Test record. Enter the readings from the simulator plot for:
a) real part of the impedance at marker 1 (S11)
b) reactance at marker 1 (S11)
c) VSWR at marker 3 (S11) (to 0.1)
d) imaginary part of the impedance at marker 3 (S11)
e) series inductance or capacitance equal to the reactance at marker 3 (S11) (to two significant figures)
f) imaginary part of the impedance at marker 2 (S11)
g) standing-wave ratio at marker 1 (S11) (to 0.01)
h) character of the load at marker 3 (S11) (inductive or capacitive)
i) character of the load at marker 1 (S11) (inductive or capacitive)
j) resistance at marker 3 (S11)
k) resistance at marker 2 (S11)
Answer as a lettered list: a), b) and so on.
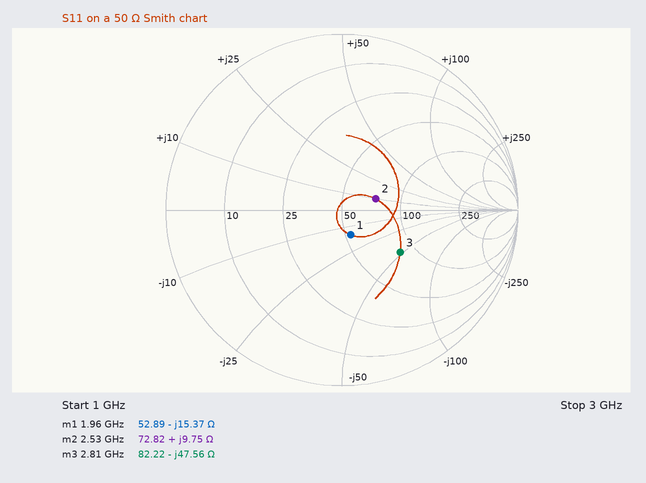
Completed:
a) 52.89 Ω
b) -15.37 Ω
c) 2.4
d) -47.56 Ω
e) 1.2 pF
f) +9.75 Ω
g) 1.35
h) capacitive
i) capacitive
j) 82.22 Ω
k) 72.82 Ω
